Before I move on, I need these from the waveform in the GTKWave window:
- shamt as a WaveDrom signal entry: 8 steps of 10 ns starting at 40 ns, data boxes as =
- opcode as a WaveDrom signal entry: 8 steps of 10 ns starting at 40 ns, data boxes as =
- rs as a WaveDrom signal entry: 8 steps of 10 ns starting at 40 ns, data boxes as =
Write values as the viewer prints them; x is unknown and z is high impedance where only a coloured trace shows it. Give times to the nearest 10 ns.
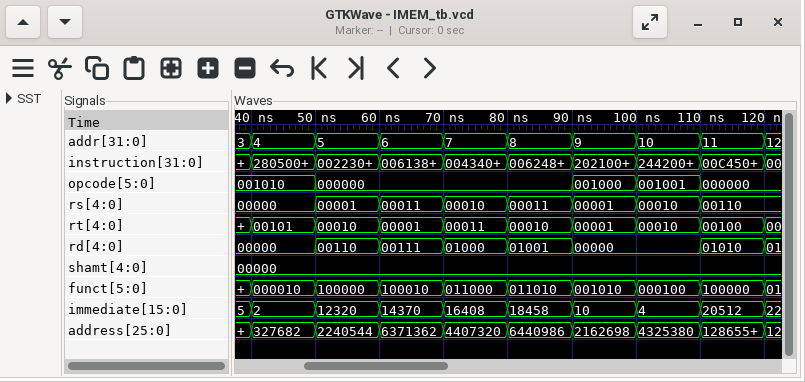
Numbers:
{name: 'shamt', wave: '=.......', data: '00000'}
{name: 'opcode', wave: '==...===', data: '001010 000000 001000 001001 000000'}
{name: 'rs', wave: '========', data: '00000 00001 00011 00010 00011 00001 00010 00110'}
